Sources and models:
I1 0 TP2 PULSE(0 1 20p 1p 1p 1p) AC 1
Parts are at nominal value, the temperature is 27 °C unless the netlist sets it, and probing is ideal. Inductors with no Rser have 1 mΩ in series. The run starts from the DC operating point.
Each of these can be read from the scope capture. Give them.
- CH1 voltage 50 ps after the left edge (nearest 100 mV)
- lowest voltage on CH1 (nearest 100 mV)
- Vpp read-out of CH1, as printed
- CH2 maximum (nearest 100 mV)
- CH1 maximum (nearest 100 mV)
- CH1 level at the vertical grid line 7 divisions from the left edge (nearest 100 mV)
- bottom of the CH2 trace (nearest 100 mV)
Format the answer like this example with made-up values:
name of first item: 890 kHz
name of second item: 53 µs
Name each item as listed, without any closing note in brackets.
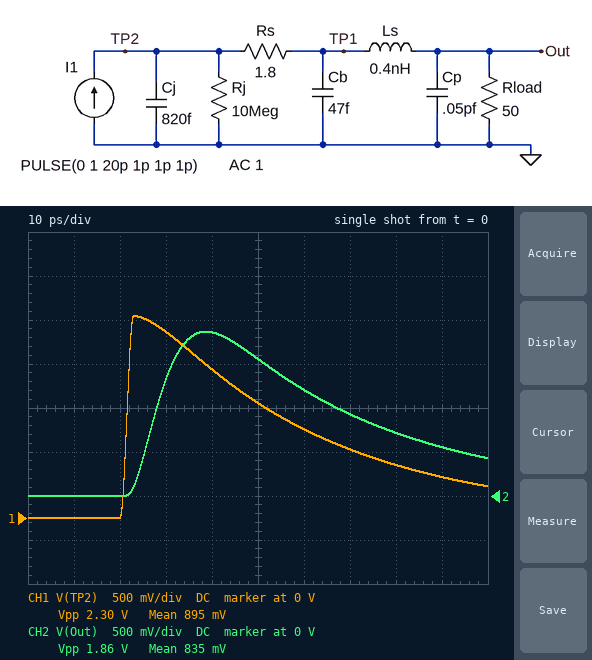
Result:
CH1 voltage 50 ps after the left edge: 1.3 V
lowest voltage on CH1: 0 V
Vpp read-out of CH1, as printed: 2.30 V
CH2 maximum: 1.9 V
CH1 maximum: 2.3 V
CH1 level at the vertical grid line 7 divisions from the left edge: 800 mV
bottom of the CH2 trace: 0 V
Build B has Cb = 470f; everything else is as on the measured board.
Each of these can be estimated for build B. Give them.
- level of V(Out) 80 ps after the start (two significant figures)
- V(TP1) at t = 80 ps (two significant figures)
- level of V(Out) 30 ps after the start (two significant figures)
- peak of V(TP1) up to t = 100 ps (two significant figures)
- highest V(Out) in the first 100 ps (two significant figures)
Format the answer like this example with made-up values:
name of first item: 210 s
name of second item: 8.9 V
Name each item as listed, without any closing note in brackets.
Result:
level of V(Out) 80 ps after the start: 730 mV
V(TP1) at t = 80 ps: 640 mV
level of V(Out) 30 ps after the start: 860 mV
peak of V(TP1) up to t = 100 ps: 1.5 V
highest V(Out) in the first 100 ps: 1.3 V
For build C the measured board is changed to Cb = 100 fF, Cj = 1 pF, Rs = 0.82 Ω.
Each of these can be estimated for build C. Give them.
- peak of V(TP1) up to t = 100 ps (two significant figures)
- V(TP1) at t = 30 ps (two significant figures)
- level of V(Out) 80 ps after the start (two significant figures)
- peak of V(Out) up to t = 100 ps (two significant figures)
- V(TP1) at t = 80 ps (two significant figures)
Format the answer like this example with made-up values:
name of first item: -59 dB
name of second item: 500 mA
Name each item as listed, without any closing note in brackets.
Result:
peak of V(TP1) up to t = 100 ps: 1.8 V
V(TP1) at t = 30 ps: 1.7 V
level of V(Out) 80 ps after the start: 740 mV
peak of V(Out) up to t = 100 ps: 1.5 V
V(TP1) at t = 80 ps: 630 mV
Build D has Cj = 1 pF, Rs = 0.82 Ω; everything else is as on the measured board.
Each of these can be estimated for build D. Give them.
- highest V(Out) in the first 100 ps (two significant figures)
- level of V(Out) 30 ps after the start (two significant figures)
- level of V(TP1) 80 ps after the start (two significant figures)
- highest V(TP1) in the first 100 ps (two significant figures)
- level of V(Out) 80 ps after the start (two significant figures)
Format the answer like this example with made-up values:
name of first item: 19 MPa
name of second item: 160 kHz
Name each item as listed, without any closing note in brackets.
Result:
highest V(Out) in the first 100 ps: 1.6 V
level of V(Out) 30 ps after the start: 1.1 V
level of V(TP1) 80 ps after the start: 620 mV
highest V(TP1) in the first 100 ps: 1.9 V
level of V(Out) 80 ps after the start: 740 mV
